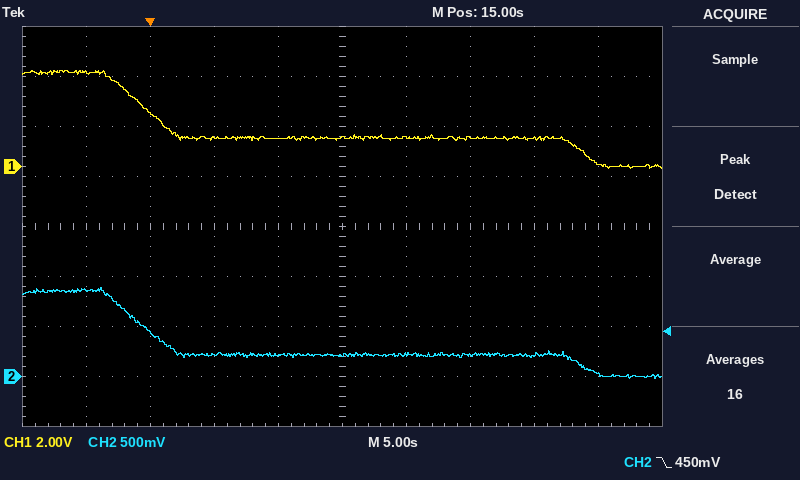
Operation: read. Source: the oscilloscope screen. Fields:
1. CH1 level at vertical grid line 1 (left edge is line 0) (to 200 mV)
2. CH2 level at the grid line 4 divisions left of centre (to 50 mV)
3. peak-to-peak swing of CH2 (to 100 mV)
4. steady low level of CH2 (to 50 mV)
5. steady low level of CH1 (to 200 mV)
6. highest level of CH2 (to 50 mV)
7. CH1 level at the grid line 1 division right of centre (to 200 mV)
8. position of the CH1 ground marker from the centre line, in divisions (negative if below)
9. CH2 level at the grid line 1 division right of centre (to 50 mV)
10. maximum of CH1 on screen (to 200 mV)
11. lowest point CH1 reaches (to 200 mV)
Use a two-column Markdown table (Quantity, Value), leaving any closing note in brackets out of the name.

| Quantity | Value |
|---|---|
| CH1 level at vertical grid line 1 (left edge is line 0) | 3.8 V |
| CH2 level at the grid line 4 divisions left of centre | 850 mV |
| peak-to-peak swing of CH2 | 900 mV |
| steady low level of CH2 | 200 mV |
| steady low level of CH1 | 1.2 V |
| highest level of CH2 | 900 mV |
| CH1 level at the grid line 1 division right of centre | 1.2 V |
| position of the CH1 ground marker from the centre line, in divisions | +1.2 div |
| CH2 level at the grid line 1 division right of centre | 200 mV |
| maximum of CH1 on screen | 3.8 V |
| lowest point CH1 reaches | 0.0 V |
